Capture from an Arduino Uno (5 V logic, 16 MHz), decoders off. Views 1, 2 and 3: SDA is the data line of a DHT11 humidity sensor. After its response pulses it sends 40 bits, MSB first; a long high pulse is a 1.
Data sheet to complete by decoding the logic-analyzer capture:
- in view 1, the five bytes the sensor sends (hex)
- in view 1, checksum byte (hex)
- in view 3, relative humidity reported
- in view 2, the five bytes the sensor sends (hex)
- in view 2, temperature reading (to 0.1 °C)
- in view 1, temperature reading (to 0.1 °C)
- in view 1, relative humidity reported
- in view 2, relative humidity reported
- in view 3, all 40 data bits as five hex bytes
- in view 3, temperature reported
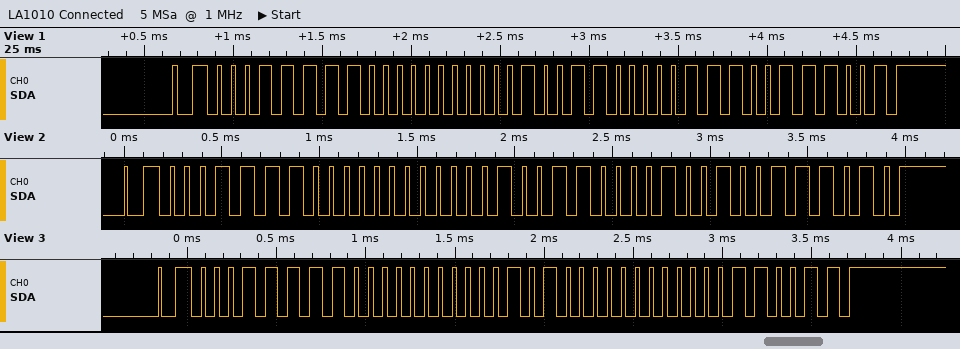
1F 00 13 07 39
0x39
31 %
1E 00 13 09 3A
19.9 °C
19.7 °C
31 %
30 %
1F 00 14 00 33
20.0 °C
